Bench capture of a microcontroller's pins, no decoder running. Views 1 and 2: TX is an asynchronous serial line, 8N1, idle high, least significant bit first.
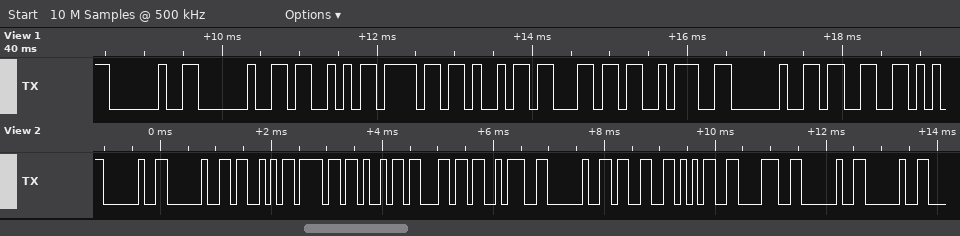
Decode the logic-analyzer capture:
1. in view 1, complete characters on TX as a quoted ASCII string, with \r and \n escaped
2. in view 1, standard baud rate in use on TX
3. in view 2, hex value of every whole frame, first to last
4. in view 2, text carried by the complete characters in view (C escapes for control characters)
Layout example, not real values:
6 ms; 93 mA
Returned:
"  Soil: 3"; 9600 baud; 0x20 0x20 0x53 0x6F 0x69 0x6C 0x3A 0x20 0x33 0x35 0x38 0x20 0x20; "  Soil: 358  "
